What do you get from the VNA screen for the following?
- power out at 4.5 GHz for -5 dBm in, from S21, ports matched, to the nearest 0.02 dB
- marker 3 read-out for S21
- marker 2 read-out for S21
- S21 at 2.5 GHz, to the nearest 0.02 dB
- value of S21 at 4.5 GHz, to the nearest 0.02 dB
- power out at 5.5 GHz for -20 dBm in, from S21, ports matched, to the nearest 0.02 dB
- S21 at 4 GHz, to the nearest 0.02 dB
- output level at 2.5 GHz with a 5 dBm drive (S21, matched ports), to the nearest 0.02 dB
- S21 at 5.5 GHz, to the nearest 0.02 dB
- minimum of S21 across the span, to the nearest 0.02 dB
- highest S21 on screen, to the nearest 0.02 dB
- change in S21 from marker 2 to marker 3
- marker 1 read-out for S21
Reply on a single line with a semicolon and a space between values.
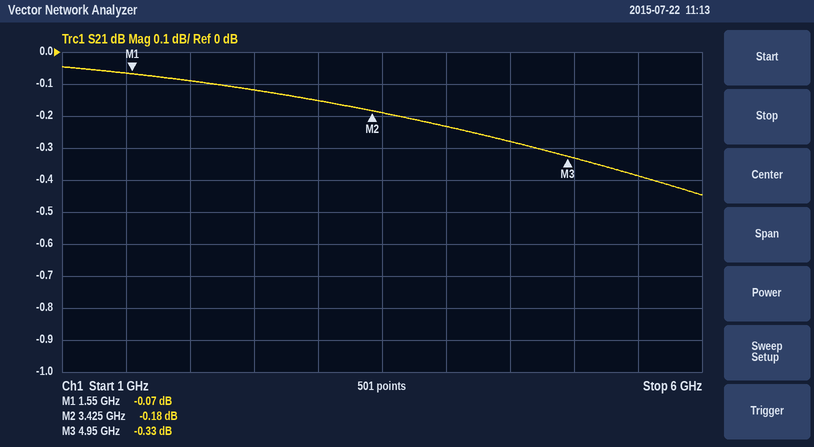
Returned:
-5.28 dBm; -0.33 dB; -0.18 dB; -0.12 dB; -0.28 dB; -20.38 dBm; -0.24 dB; 4.88 dBm; -0.38 dB; -0.44 dB; -0.04 dB; -0.15 dB; -0.07 dB
